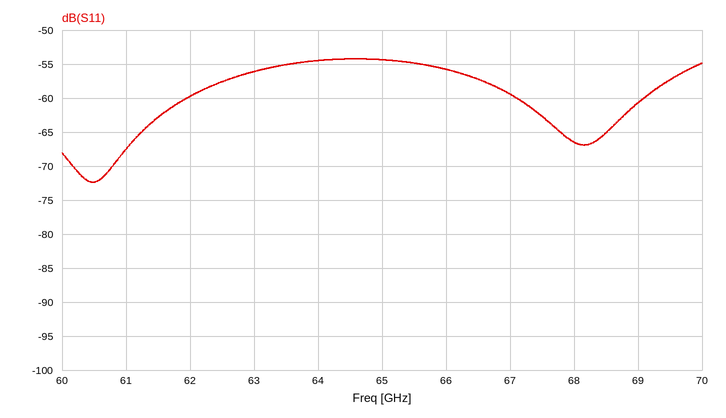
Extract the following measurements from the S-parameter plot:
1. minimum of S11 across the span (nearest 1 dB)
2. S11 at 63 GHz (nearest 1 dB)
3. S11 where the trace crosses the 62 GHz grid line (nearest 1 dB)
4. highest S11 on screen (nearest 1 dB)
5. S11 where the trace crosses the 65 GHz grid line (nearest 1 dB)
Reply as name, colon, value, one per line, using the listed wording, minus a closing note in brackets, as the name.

minimum of S11 across the span: -72 dB
S11 at 63 GHz: -56 dB
S11 where the trace crosses the 62 GHz grid line: -60 dB
highest S11 on screen: -54 dB
S11 where the trace crosses the 65 GHz grid line: -54 dB
